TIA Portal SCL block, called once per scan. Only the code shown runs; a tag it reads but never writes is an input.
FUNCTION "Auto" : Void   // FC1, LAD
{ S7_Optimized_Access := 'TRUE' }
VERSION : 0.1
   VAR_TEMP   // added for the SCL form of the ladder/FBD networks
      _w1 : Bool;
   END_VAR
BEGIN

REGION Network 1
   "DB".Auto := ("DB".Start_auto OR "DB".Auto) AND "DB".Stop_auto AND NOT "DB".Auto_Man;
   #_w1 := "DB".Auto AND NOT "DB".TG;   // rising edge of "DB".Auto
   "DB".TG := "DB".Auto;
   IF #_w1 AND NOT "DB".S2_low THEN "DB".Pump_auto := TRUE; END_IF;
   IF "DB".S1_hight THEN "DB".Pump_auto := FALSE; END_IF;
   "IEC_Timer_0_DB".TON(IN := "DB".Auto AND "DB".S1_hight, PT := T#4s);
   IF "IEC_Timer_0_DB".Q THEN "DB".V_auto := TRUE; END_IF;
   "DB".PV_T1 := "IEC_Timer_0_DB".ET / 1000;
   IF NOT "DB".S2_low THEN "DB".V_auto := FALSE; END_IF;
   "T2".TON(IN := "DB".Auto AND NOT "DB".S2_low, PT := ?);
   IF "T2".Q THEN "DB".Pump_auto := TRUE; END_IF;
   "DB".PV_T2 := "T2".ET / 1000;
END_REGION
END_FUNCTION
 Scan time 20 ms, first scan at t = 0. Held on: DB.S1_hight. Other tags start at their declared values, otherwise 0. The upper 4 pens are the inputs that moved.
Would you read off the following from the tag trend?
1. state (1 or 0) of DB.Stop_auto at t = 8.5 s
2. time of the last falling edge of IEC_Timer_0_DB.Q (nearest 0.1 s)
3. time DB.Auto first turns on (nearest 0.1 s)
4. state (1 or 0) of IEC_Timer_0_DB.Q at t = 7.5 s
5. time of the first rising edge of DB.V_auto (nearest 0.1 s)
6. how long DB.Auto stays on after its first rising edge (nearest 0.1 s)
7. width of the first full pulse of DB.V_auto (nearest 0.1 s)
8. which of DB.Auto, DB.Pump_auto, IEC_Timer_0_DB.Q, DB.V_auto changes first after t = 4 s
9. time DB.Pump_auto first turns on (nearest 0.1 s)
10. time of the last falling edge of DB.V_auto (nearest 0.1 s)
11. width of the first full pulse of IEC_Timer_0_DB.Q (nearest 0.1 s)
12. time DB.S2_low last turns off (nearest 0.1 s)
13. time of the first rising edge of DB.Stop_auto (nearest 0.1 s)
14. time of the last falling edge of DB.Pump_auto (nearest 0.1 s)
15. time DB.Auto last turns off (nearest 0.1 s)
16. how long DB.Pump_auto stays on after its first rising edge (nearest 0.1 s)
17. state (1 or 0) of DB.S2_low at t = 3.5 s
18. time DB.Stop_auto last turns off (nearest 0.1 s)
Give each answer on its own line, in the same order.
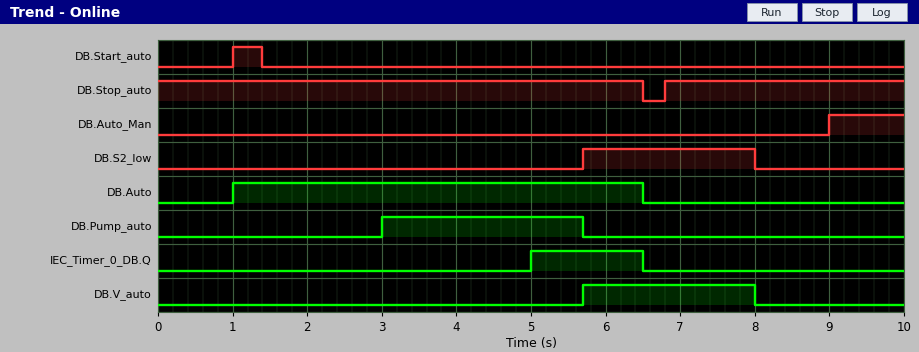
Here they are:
1
6.5 s
1.0 s
0
5.7 s
5.5 s
2.3 s
IEC_Timer_0_DB.Q
3.0 s
8.0 s
1.5 s
8.0 s
6.8 s
5.7 s
6.5 s
2.7 s
0
6.5 s
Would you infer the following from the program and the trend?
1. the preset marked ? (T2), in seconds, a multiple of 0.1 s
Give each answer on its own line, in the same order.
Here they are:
2.0 s
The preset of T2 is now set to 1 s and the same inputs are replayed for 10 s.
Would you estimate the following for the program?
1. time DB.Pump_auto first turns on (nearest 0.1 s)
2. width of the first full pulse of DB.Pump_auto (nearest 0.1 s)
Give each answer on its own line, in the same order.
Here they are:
2.0 s
3.7 s
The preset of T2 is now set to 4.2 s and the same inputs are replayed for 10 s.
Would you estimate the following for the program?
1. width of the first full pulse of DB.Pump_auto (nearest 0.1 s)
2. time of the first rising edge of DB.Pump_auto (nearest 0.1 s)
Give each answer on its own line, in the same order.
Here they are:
0.5 s
5.2 s
